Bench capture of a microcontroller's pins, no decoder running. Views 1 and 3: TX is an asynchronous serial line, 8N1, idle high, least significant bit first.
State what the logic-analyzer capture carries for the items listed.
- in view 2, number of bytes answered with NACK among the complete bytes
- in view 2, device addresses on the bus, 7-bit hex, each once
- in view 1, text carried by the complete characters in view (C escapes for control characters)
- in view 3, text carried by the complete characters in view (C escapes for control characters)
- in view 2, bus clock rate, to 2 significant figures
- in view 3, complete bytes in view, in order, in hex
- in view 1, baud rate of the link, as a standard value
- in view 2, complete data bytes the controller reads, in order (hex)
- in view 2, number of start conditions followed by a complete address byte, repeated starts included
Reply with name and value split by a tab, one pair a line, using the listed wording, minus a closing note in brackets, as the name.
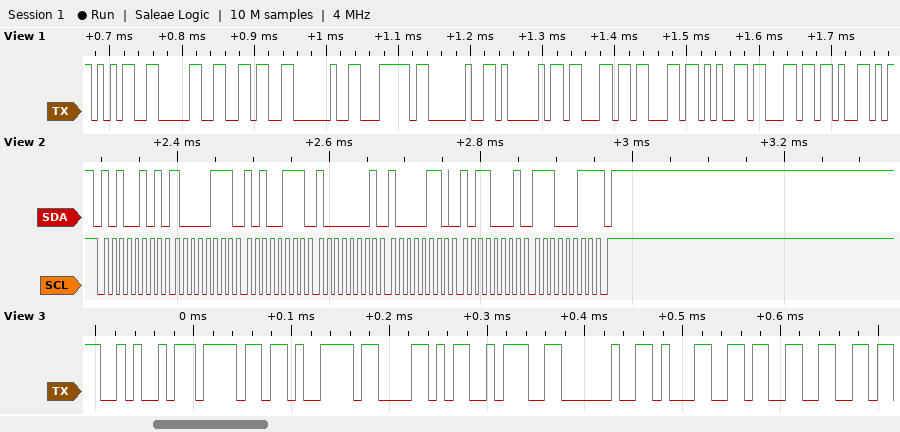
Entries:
in view 2, number of bytes answered with NACK among the complete bytes	1
in view 2, device addresses on the bus, 7-bit hex, each once	0x52
in view 1, text carried by the complete characters in view	"506 | AccelY"
in view 3, text carried by the complete characters in view	"JoyX: 13"
in view 2, bus clock rate, to 2 significant figures	100 kHz
in view 3, complete bytes in view, in order, in hex	4A 6F 79 58 3A 20 31 33
in view 1, baud rate of the link, as a standard value	115200 baud
in view 2, complete data bytes the controller reads, in order	87 A7 81 86 B1 E3
in view 2, number of start conditions followed by a complete address byte, repeated starts included	1
